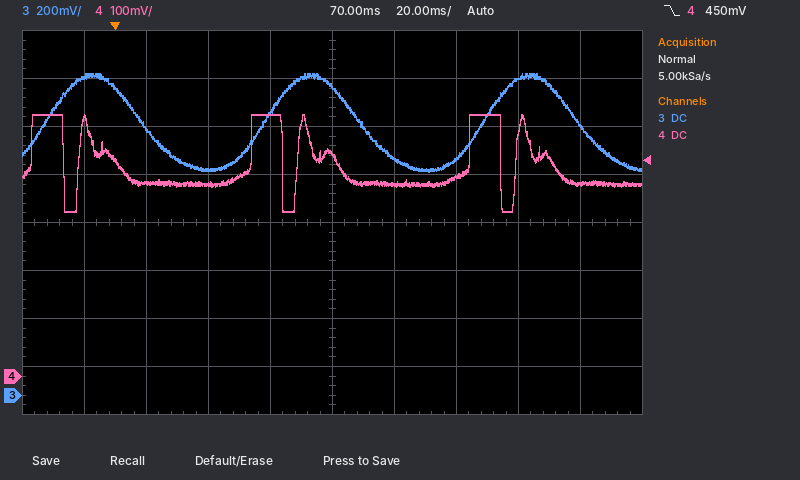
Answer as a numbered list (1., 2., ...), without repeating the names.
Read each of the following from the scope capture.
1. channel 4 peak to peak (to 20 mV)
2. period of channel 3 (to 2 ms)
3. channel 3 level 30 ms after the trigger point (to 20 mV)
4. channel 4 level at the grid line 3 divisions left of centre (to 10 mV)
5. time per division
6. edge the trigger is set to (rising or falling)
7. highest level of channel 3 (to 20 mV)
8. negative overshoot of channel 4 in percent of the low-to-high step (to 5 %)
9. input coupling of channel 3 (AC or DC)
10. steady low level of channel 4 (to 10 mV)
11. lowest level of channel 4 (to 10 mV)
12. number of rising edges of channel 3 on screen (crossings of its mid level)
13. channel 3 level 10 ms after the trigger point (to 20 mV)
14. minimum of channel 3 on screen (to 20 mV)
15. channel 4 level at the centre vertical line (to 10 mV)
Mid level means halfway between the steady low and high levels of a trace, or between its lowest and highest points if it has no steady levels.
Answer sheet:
1. 200 mV
2. 70 ms
3. 940 mV
4. 400 mV
5. 20 ms
6. falling
7. 1.34 V
8. 40 %
9. DC
10. 400 mV
11. 340 mV
12. 3
13. 1.12 V
14. 940 mV
15. 460 mV
